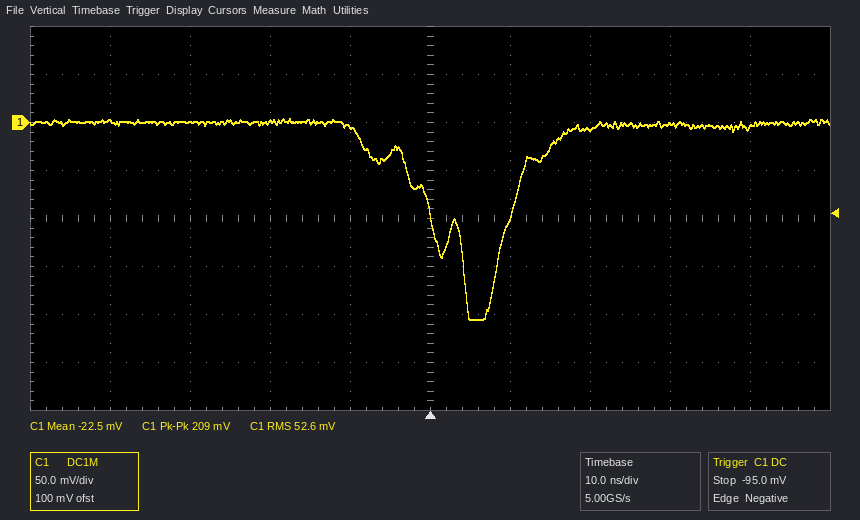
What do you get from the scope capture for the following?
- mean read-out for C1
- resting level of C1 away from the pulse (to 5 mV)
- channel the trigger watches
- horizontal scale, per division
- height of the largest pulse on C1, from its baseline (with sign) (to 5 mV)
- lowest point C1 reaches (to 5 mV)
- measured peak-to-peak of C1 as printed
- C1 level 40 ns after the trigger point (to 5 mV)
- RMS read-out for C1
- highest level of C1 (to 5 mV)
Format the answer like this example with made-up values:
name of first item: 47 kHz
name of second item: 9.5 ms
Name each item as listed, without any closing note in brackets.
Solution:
mean read-out for C1: -22.5 mV
resting level of C1 away from the pulse: 0 mV
channel the trigger watches: C1
horizontal scale, per division: 10 ns
height of the largest pulse on C1, from its baseline (with sign): -205 mV
lowest point C1 reaches: -205 mV
measured peak-to-peak of C1 as printed: 209 mV
C1 level 40 ns after the trigger point: -5 mV
RMS read-out for C1: 52.6 mV
highest level of C1: 5 mV
